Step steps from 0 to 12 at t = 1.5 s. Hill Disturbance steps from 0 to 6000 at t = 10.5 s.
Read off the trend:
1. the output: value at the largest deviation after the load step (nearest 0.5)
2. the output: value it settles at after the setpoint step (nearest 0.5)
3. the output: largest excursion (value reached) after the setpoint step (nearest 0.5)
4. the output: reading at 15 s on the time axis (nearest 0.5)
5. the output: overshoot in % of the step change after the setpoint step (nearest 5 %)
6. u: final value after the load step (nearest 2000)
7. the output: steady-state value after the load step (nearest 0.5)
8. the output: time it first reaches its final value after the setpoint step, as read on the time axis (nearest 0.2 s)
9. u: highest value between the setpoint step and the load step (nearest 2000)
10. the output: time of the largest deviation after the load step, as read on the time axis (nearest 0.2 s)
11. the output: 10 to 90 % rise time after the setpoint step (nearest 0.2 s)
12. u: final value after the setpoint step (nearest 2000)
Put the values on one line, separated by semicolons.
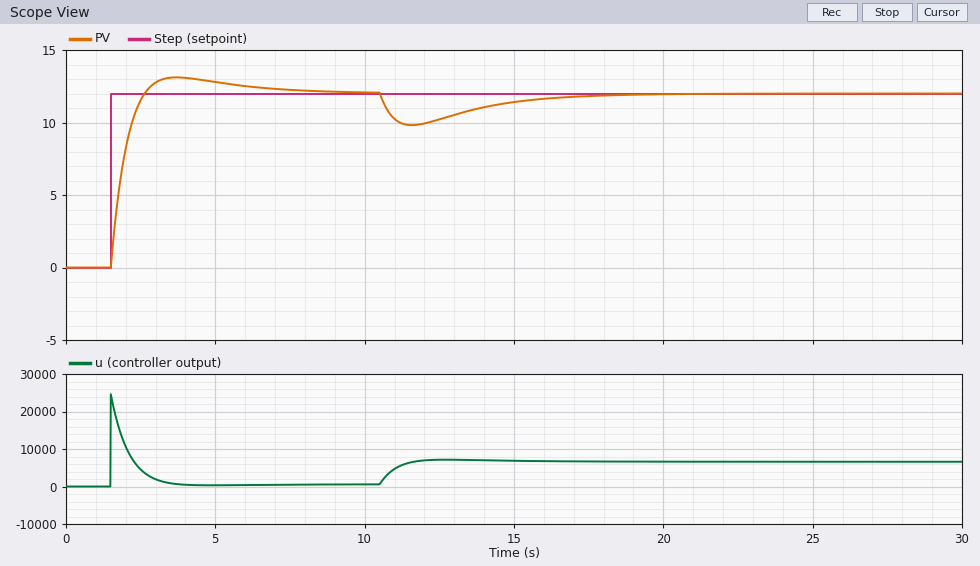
10.0; 12.0; 13.0; 11.5; 10 %; 6000; 12.0; 2.6 s; 24000; 11.6 s; 0.8 s; 0
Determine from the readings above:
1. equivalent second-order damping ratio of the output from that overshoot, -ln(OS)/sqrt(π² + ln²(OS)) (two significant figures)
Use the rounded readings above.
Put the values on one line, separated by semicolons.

0.59
